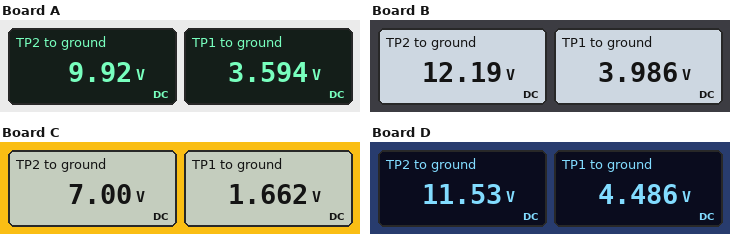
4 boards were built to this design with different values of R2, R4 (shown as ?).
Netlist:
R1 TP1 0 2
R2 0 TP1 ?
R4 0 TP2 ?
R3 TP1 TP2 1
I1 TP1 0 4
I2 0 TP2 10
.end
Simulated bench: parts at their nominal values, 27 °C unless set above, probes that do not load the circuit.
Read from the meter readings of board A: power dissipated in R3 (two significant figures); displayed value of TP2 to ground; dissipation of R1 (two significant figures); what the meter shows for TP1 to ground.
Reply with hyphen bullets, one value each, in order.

- 40 W
- 9.92 V
- 6.5 W
- 3.594 V
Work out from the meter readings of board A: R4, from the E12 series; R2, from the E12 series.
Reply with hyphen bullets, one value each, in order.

- 2.7 Ω
- 6.8 Ω
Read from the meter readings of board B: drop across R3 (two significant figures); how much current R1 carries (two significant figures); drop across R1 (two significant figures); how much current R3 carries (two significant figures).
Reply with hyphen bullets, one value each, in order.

- 8.2 V
- 2.0 A
- 4.0 V
- 8.2 A
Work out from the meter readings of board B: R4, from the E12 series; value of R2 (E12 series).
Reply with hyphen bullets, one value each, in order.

- 6.8 Ω
- 1.8 Ω
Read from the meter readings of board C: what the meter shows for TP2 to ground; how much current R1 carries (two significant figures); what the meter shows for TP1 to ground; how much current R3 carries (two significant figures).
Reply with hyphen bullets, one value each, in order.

- 7.00 V
- 830 mA
- 1.662 V
- 5.3 A
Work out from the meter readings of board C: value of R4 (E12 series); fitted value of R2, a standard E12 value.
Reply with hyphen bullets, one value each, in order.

- 1.5 Ω
- 3.3 Ω
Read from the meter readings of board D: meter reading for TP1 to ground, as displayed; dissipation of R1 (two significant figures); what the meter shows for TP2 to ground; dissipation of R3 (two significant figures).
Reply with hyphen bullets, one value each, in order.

- 4.486 V
- 10 W
- 11.53 V
- 50 W
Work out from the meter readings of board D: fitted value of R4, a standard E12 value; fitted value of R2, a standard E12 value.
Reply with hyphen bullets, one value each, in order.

- 3.9 Ω
- 5.6 Ω
